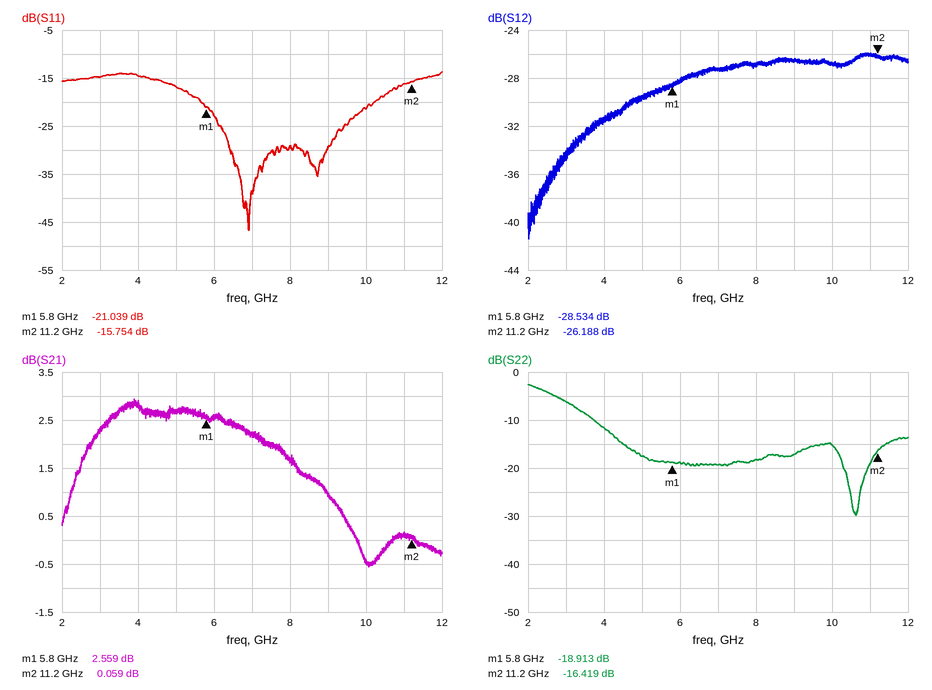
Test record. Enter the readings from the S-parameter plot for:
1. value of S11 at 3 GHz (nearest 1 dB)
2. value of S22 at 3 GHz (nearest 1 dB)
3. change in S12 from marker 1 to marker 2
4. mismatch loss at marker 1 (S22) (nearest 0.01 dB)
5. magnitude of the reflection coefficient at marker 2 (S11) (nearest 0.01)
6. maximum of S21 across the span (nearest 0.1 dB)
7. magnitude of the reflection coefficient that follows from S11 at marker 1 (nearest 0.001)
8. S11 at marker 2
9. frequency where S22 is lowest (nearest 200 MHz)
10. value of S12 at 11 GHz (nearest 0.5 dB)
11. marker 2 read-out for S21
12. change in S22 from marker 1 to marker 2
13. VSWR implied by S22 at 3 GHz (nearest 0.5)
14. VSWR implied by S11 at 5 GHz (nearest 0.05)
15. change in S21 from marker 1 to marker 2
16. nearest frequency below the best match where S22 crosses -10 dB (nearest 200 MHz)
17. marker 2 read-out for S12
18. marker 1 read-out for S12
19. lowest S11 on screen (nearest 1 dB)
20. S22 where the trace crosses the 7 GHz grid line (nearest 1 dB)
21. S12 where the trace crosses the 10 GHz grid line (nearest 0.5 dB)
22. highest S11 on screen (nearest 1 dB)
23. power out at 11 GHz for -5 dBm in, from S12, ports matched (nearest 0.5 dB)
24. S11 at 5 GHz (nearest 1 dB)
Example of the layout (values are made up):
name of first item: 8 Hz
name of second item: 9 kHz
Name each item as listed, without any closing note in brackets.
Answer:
value of S11 at 3 GHz: -15 dB
value of S22 at 3 GHz: -6 dB
change in S12 from marker 1 to marker 2: 2.346 dB
mismatch loss at marker 1 (S22): 0.06 dB
magnitude of the reflection coefficient at marker 2 (S11): 0.16
maximum of S21 across the span: 2.9 dB
magnitude of the reflection coefficient that follows from S11 at marker 1: 0.089
S11 at marker 2: -15.754 dB
frequency where S22 is lowest: 10.6 GHz
value of S12 at 11 GHz: -26.0 dB
marker 2 read-out for S21: 0.059 dB
change in S22 from marker 1 to marker 2: 2.494 dB
VSWR implied by S22 at 3 GHz: 3.0
VSWR implied by S11 at 5 GHz: 1.35
change in S21 from marker 1 to marker 2: -2.500 dB
nearest frequency below the best match where S22 crosses -10 dB: 3.8 GHz
marker 2 read-out for S12: -26.188 dB
marker 1 read-out for S12: -28.534 dB
lowest S11 on screen: -47 dB
S22 where the trace crosses the 7 GHz grid line: -19 dB
S12 where the trace crosses the 10 GHz grid line: -27.0 dB
highest S11 on screen: -14 dB
power out at 11 GHz for -5 dBm in, from S12, ports matched: -31.0 dBm
S11 at 5 GHz: -17 dB
